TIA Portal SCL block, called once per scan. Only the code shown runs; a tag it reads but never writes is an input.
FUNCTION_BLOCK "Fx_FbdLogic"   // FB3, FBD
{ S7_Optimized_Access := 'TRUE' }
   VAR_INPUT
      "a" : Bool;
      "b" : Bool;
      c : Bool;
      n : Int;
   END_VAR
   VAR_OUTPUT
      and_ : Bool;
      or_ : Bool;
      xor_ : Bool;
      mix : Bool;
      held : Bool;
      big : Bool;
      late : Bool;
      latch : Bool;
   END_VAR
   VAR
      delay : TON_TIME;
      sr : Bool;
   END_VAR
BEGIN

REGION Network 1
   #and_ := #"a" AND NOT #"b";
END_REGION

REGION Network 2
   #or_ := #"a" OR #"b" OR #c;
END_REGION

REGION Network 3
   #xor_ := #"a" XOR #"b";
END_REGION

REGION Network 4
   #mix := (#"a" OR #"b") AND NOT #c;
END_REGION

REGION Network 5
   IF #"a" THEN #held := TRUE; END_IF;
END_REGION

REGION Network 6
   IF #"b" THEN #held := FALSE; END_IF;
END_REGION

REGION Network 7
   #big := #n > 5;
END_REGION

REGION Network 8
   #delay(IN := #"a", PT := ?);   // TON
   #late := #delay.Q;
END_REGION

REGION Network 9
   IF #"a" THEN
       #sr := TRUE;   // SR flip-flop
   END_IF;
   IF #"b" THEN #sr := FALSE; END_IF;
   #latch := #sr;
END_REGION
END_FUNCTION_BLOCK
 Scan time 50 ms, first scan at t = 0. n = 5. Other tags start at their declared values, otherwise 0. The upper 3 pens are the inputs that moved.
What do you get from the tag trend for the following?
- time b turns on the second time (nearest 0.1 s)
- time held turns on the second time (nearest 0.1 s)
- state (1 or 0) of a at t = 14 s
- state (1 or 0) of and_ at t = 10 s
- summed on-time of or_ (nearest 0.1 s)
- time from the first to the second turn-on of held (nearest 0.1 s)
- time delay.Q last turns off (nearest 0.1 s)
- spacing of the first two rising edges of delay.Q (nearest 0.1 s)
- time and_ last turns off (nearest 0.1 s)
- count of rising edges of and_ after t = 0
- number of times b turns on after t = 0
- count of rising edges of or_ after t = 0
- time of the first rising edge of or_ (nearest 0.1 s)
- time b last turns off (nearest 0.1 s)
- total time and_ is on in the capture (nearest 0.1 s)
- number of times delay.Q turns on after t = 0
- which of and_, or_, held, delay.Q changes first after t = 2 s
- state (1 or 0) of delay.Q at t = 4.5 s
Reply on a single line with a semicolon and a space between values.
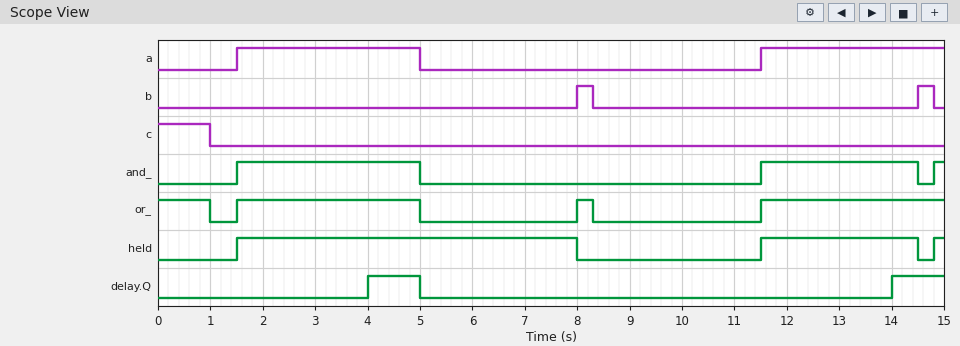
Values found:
14.5 s; 11.5 s; 1; 0; 8.3 s; 10.0 s; 5.0 s; 10.0 s; 14.5 s; 3; 2; 3; 1.5 s; 14.8 s; 6.7 s; 2; delay.Q; 1
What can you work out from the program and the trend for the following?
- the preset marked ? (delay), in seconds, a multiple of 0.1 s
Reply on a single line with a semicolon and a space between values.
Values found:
2.5 s
